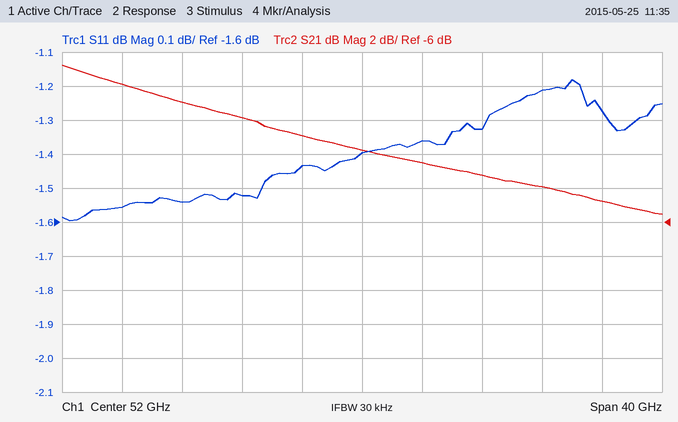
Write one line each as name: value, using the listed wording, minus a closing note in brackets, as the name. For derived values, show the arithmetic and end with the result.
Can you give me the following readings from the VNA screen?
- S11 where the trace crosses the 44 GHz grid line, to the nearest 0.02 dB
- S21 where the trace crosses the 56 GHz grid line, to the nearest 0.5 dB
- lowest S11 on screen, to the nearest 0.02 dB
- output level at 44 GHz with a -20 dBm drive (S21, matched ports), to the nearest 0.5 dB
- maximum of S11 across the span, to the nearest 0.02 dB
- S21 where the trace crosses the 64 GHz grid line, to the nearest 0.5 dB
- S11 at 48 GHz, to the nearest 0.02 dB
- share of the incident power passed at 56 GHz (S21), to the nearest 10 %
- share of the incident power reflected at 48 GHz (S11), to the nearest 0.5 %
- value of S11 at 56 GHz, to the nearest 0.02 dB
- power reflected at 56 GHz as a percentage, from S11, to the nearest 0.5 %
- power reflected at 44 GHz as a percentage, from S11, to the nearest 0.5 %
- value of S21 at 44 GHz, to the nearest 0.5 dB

S11 where the trace crosses the 44 GHz grid line, to the nearest 0.02 dB: -1.52 dB
S21 where the trace crosses the 56 GHz grid line, to the nearest 0.5 dB: -2.5 dB
lowest S11 on screen, to the nearest 0.02 dB: -1.60 dB
output level at 44 GHz with a -20 dBm drive (S21, matched ports), to the nearest 0.5 dB: -20 dBm + (0.0 dB) = -20.0 dBm
maximum of S11 across the span, to the nearest 0.02 dB: -1.18 dB
S21 where the trace crosses the 64 GHz grid line, to the nearest 0.5 dB: -4.0 dB
S11 at 48 GHz, to the nearest 0.02 dB: -1.44 dB
share of the incident power passed at 56 GHz (S21), to the nearest 10 %: 10^(-2.5/10) ≈ 56.2 %, so 60 % to the nearest 10 %
share of the incident power reflected at 48 GHz (S11), to the nearest 0.5 %: 10^(-1.44/10) ≈ 71.8 %, so 72.0 % to the nearest 0.5 %
value of S11 at 56 GHz, to the nearest 0.02 dB: -1.36 dB
power reflected at 56 GHz as a percentage, from S11, to the nearest 0.5 %: 10^(-1.36/10) ≈ 73.1 %, so 73.0 % to the nearest 0.5 %
power reflected at 44 GHz as a percentage, from S11, to the nearest 0.5 %: 10^(-1.52/10) ≈ 70.5 %
value of S21 at 44 GHz, to the nearest 0.5 dB: 0.0 dB
